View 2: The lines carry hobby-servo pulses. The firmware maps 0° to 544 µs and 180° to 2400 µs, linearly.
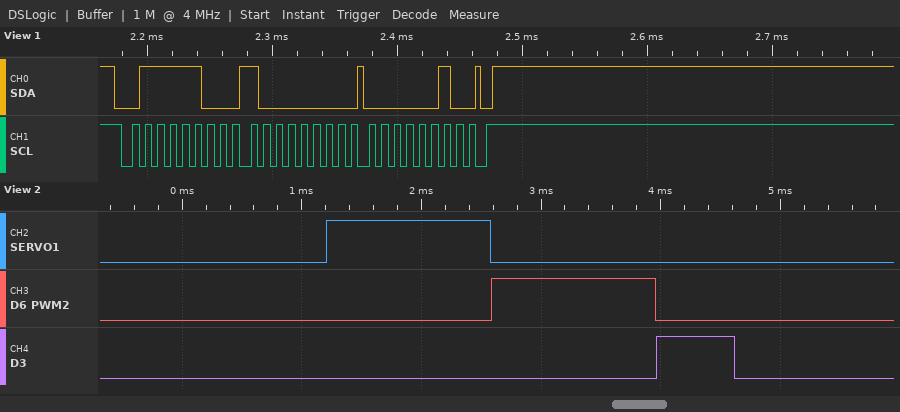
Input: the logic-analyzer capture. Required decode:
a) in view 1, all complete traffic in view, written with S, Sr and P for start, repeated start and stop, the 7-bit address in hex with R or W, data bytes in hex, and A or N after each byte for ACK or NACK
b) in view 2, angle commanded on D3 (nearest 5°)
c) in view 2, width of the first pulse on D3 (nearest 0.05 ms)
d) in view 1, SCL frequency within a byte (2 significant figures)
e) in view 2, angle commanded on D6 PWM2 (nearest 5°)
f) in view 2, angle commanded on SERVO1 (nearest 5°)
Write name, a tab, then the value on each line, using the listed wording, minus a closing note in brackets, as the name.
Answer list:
in view 1, all complete traffic in view, written with S, Sr and P for start, repeated start and stop, the 7-bit address in hex with R or W, data bytes in hex, and A or N after each byte for ACK or NACK	S 3EW A 80 A 02 A P
in view 2, angle commanded on D3	10°
in view 2, width of the first pulse on D3	0.65 ms
in view 1, SCL frequency within a byte	100 kHz
in view 2, angle commanded on D6 PWM2	80°
in view 2, angle commanded on SERVO1	80°
